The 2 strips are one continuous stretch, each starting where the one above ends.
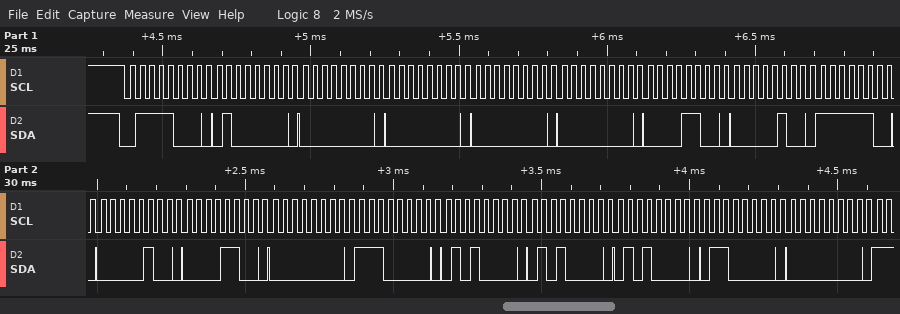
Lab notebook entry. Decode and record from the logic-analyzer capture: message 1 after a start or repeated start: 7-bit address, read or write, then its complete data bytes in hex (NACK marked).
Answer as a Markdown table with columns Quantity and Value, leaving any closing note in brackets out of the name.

| Quantity | Value |
|---|---|
| message 1 after a start or repeated start: 7-bit address, read or write, then its complete data bytes in hex | 0x3C write: 40 00 00 00 00 0C 04 FC 04 0C 00 E0 50 50 50 60 00 |
